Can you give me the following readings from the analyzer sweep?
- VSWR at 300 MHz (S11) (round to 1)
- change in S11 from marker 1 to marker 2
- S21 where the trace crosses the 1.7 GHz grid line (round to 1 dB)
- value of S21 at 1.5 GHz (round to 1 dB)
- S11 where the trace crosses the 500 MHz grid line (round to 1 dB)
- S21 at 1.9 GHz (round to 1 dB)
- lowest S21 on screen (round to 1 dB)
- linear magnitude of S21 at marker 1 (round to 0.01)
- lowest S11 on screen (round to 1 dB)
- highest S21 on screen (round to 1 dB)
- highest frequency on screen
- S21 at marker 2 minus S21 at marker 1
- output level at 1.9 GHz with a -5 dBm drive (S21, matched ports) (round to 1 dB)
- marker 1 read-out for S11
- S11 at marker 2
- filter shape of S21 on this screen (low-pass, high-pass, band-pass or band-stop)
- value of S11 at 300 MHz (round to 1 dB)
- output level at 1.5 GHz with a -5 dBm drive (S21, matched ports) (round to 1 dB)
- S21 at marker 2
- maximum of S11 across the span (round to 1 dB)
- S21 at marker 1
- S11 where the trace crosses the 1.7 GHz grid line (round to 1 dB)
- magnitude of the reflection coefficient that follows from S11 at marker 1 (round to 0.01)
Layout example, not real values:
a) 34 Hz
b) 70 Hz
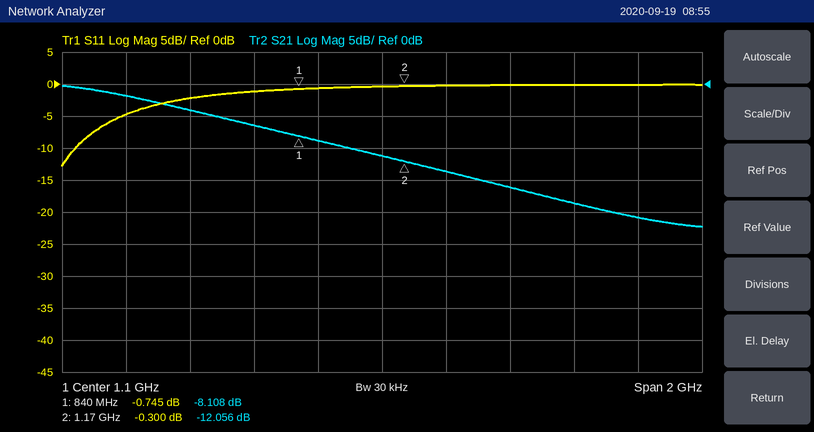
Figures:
a) 4
b) 0.445 dB
c) -19 dB
d) -16 dB
e) -2 dB
f) -21 dB
g) -22 dB
h) 0.39
i) -13 dB
j) 0 dB
k) 2.1 GHz
l) -3.948 dB
m) -26 dBm
n) -0.745 dB
o) -0.300 dB
p) low-pass
q) -5 dB
r) -21 dBm
s) -12.056 dB
t) 0 dB
u) -8.108 dB
v) 0 dB
w) 0.92
